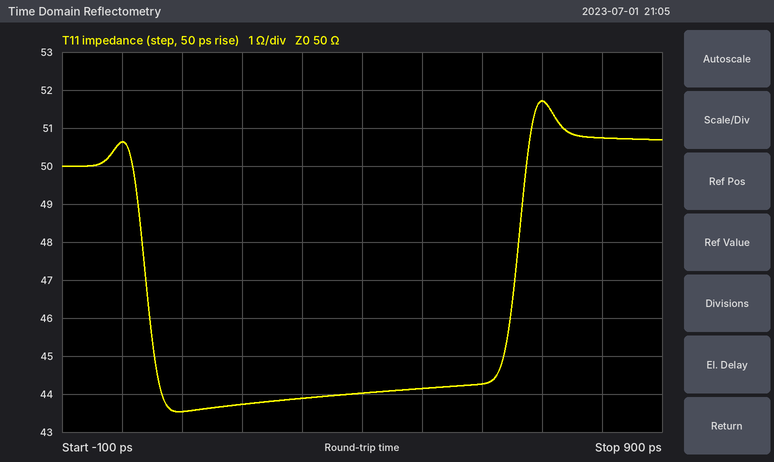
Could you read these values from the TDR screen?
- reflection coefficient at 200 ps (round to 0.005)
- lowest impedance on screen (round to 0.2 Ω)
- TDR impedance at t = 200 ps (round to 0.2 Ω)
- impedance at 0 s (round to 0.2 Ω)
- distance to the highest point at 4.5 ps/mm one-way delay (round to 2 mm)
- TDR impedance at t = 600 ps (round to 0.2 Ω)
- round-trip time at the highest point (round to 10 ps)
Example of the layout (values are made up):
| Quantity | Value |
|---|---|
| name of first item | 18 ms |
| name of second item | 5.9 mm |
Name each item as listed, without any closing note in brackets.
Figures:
| Quantity | Value |
|---|---|
| reflection coefficient at 200 ps | -0.065 |
| lowest impedance on screen | 43.6 Ω |
| TDR impedance at t = 200 ps | 43.8 Ω |
| impedance at 0 s | 50.6 Ω |
| distance to the highest point at 4.5 ps/mm one-way delay | 78 mm |
| TDR impedance at t = 600 ps | 44.2 Ω |
| round-trip time at the highest point | 700 ps |
